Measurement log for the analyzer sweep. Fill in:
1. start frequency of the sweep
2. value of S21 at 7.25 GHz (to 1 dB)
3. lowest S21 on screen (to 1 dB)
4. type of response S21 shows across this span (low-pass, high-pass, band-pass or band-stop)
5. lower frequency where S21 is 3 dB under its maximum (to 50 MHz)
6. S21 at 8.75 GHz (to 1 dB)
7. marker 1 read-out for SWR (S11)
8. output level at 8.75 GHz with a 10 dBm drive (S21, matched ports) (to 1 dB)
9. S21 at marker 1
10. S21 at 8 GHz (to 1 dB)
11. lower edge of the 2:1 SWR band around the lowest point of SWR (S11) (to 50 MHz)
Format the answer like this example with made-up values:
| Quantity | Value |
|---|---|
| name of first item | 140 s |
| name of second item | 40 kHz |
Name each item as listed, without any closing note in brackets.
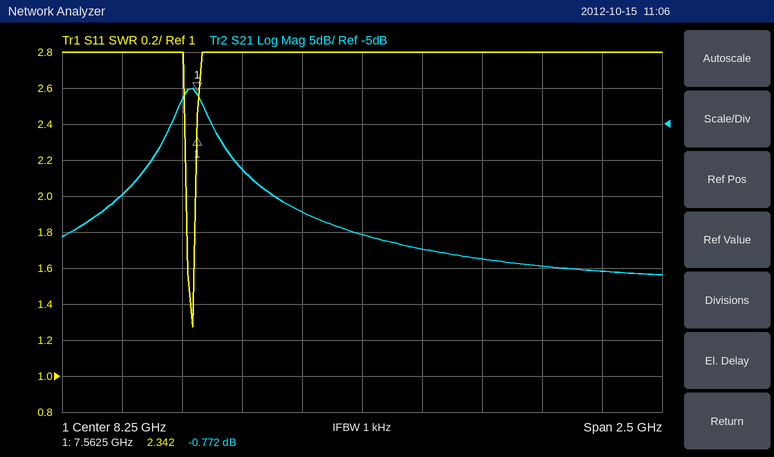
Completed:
| Quantity | Value |
|---|---|
| start frequency of the sweep | 7 GHz |
| value of S21 at 7.25 GHz | -15 dB |
| lowest S21 on screen | -26 dB |
| type of response S21 shows across this span | band-pass |
| lower frequency where S21 is 3 dB under its maximum | 7.50 GHz |
| S21 at 8.75 GHz | -24 dB |
| marker 1 read-out for SWR | 2.342 |
| output level at 8.75 GHz with a 10 dBm drive (S21, matched ports) | -14 dBm |
| S21 at marker 1 | -0.772 dB |
| S21 at 8 GHz | -17 dB |
| lower edge of the 2:1 SWR band around the lowest point of SWR (S11) | 7.50 GHz |
